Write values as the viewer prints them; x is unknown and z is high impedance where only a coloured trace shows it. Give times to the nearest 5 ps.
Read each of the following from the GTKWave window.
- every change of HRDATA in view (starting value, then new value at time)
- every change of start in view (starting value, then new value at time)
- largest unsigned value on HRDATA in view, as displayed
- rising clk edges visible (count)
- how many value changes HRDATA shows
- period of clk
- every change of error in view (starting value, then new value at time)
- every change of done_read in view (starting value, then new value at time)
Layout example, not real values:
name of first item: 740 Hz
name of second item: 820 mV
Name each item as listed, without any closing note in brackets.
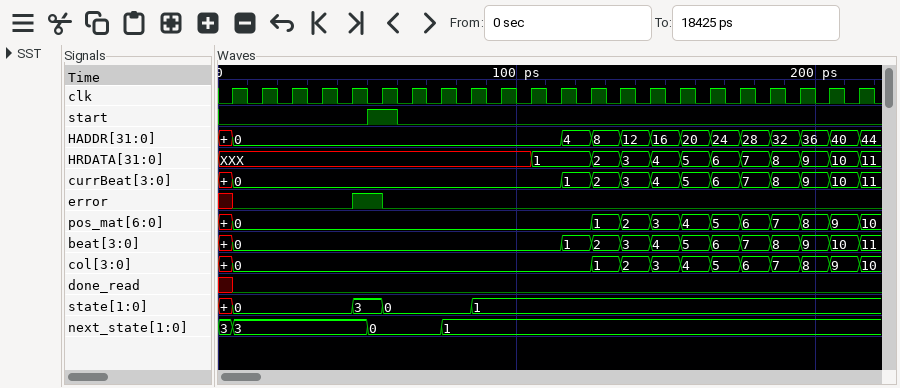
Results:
every change of HRDATA in view: XXX, 1 at 105 ps, 2 at 125 ps, 3 at 135 ps, 4 at 145 ps, 5 at 155 ps, 6 at 165 ps, 7 at 175 ps, 8 at 185 ps, 9 at 195 ps, 10 at 205 ps, 11 at 215 ps
every change of start in view: 0, 1 at 50 ps, 0 at 60 ps
largest unsigned value on HRDATA in view, as displayed: 11
rising clk edges visible: 22
how many value changes HRDATA shows: 11
period of clk: 10 ps
every change of error in view: x, 0 at 5 ps, 1 at 45 ps, 0 at 55 ps
every change of done_read in view: x, 0 at 5 ps
